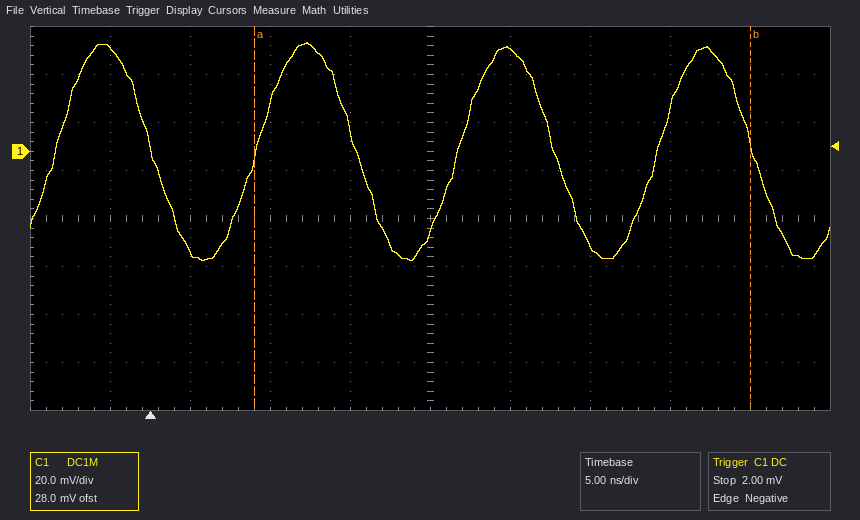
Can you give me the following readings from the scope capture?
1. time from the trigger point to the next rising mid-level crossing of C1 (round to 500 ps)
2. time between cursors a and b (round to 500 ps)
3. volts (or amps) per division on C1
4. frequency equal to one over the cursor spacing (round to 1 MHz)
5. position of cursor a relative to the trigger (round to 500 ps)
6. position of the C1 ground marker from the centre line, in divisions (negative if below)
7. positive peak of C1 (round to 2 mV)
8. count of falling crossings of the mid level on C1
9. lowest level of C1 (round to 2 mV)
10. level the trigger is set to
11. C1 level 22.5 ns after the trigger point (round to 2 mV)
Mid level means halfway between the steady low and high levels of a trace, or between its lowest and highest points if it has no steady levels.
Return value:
6.5 ns
31.0 ns
20 mV
32 MHz
+6.5 ns
+1.4 div
46 mV
4
-46 mV
2.00 mV
42 mV
